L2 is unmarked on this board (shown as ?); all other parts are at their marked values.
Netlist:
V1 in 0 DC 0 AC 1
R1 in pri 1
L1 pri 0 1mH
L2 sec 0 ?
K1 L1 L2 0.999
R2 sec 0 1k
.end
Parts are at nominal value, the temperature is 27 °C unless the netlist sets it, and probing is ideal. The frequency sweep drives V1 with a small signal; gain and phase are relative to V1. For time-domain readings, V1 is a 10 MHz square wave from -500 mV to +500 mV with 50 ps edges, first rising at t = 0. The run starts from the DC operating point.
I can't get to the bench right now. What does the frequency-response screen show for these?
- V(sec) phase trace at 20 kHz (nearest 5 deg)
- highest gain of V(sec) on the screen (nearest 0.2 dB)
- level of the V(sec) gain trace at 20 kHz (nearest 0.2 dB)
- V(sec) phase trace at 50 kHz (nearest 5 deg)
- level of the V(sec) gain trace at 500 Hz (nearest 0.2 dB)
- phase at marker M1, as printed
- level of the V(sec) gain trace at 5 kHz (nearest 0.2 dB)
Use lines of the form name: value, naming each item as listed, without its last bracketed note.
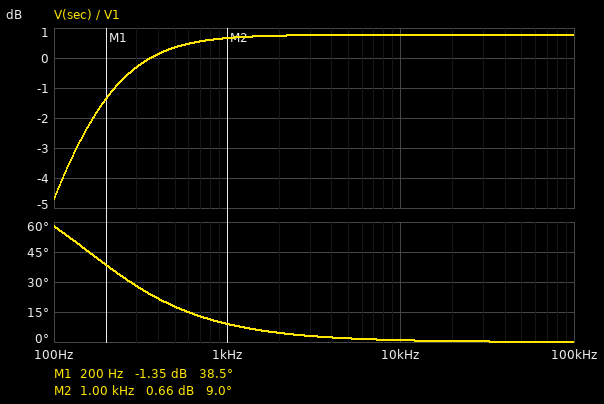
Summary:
V(sec) phase trace at 20 kHz: 0 deg
highest gain of V(sec) on the screen: 0.8 dB
level of the V(sec) gain trace at 20 kHz: 0.8 dB
V(sec) phase trace at 50 kHz: 0 deg
level of the V(sec) gain trace at 500 Hz: 0.4 dB
phase at marker M1, as printed: 38.5 deg
level of the V(sec) gain trace at 5 kHz: 0.8 dB
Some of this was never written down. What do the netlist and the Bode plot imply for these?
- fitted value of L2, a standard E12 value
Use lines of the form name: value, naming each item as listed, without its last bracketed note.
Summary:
fitted value of L2, a standard E12 value: 1.2 mH
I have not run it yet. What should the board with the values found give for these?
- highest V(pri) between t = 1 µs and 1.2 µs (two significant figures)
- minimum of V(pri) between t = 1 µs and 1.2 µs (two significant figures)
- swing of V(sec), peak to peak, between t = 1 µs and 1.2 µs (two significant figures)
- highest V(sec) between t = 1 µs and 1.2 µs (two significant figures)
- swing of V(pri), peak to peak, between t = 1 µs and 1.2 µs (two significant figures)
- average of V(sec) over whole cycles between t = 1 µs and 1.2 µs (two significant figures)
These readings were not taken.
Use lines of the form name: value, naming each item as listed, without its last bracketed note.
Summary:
highest V(pri) between t = 1 µs and 1.2 µs: 1.0 V
minimum of V(pri) between t = 1 µs and 1.2 µs: -1.8 mV
swing of V(sec), peak to peak, between t = 1 µs and 1.2 µs: 1.1 V
highest V(sec) between t = 1 µs and 1.2 µs: 1.1 V
swing of V(pri), peak to peak, between t = 1 µs and 1.2 µs: 1.0 V
average of V(sec) over whole cycles between t = 1 µs and 1.2 µs: 550 mV
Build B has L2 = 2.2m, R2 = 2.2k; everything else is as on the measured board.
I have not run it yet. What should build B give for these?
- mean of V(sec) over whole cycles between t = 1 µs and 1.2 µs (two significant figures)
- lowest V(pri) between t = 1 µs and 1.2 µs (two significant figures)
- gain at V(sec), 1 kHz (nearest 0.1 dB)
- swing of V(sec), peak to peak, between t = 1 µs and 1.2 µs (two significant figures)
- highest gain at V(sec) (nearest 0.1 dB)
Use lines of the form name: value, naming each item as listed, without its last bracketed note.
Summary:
mean of V(sec) over whole cycles between t = 1 µs and 1.2 µs: 740 mV
lowest V(pri) between t = 1 µs and 1.2 µs: -1.6 mV
gain at V(sec), 1 kHz: 3.3 dB
swing of V(sec), peak to peak, between t = 1 µs and 1.2 µs: 1.5 V
highest gain at V(sec): 3.4 dB
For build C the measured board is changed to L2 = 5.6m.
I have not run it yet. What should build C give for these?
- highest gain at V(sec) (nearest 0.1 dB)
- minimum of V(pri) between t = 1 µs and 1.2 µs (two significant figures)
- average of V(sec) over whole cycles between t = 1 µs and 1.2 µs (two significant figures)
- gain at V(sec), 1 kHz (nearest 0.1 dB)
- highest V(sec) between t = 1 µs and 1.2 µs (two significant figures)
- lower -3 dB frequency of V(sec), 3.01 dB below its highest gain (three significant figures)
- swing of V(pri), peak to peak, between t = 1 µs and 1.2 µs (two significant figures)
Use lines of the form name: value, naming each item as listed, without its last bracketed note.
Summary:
highest gain at V(sec): 7.4 dB
minimum of V(pri) between t = 1 µs and 1.2 µs: -6.1 mV
average of V(sec) over whole cycles between t = 1 µs and 1.2 µs: 1.2 V
gain at V(sec), 1 kHz: 7.3 dB
highest V(sec) between t = 1 µs and 1.2 µs: 2.3 V
lower -3 dB frequency of V(sec), 3.01 dB below its highest gain: 158 Hz
swing of V(pri), peak to peak, between t = 1 µs and 1.2 µs: 1.0 V
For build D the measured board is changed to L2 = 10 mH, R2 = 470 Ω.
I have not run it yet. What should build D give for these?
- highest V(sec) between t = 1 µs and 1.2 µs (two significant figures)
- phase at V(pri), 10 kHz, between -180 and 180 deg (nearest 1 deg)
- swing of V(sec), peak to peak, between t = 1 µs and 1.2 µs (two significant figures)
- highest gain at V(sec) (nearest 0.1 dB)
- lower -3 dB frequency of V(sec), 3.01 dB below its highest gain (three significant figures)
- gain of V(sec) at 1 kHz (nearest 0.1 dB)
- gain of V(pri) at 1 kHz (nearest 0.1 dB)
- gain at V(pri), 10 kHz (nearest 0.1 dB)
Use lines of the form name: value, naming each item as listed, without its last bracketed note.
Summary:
highest V(sec) between t = 1 µs and 1.2 µs: 2.4 V
phase at V(pri), 10 kHz, between -180 and 180 deg: 1 deg
swing of V(sec), peak to peak, between t = 1 µs and 1.2 µs: 1.7 V
highest gain at V(sec): 9.8 dB
lower -3 dB frequency of V(sec), 3.01 dB below its highest gain: 156 Hz
gain of V(sec) at 1 kHz: 9.7 dB
gain of V(pri) at 1 kHz: -0.3 dB
gain at V(pri), 10 kHz: -0.2 dB
